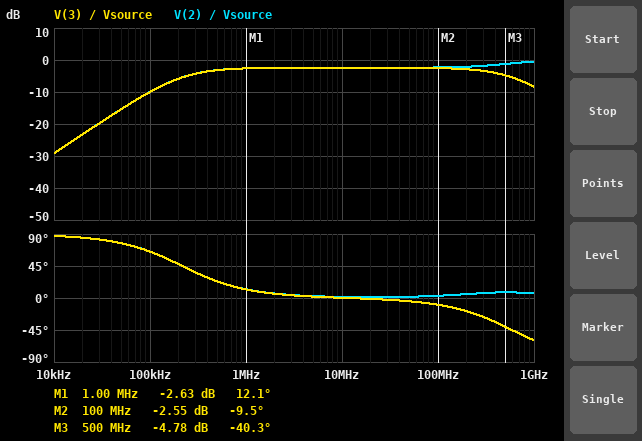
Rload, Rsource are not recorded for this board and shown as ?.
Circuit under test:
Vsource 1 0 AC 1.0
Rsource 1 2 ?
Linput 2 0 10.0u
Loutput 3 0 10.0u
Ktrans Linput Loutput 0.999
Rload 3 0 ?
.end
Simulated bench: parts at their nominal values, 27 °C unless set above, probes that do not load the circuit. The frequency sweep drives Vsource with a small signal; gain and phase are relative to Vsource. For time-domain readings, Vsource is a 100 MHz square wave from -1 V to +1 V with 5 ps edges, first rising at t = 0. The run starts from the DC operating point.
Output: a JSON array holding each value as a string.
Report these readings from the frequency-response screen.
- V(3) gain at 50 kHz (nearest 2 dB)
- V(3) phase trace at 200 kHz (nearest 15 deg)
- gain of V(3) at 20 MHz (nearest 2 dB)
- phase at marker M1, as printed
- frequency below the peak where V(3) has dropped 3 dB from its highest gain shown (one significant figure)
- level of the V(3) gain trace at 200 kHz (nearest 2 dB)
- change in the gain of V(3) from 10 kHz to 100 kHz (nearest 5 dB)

["-16 dB", "45 deg", "-2 dB", "12.1 deg", "200 kHz", "-6 dB", "20 dB"]
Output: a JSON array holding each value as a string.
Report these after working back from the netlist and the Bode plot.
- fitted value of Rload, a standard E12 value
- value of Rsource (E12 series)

["56 Ω", "18 Ω"]
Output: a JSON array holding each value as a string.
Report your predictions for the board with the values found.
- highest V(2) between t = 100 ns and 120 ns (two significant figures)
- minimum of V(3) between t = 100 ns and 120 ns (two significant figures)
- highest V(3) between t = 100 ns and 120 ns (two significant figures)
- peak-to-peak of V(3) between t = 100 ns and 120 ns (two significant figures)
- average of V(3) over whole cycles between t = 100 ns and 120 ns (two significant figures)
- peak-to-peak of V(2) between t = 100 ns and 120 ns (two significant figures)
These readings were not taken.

["1.9 V", "-110 mV", "1.4 V", "1.5 V", "650 mV", "2.5 V"]
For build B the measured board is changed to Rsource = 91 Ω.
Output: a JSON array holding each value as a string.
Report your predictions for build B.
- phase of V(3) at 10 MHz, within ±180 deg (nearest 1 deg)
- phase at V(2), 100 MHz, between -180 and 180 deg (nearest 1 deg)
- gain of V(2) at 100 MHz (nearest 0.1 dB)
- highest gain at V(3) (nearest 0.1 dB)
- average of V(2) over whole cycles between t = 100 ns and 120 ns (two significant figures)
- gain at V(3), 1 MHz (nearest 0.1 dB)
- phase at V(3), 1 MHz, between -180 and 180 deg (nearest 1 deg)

["3 deg", "8 deg", "-8.2 dB", "-8.4 dB", "260 mV", "-9.5 dB", "29 deg"]
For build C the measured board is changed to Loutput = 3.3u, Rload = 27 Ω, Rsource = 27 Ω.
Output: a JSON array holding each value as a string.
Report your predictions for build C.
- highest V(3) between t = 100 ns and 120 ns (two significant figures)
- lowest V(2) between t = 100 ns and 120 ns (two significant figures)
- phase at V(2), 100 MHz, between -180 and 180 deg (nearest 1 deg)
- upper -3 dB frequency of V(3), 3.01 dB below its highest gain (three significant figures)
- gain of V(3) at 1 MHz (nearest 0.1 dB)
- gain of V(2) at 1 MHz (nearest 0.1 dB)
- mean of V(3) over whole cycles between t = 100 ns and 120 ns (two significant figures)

["780 mV", "-650 mV", "2 deg", "867 MHz", "-7.7 dB", "-2.9 dB", "350 mV"]
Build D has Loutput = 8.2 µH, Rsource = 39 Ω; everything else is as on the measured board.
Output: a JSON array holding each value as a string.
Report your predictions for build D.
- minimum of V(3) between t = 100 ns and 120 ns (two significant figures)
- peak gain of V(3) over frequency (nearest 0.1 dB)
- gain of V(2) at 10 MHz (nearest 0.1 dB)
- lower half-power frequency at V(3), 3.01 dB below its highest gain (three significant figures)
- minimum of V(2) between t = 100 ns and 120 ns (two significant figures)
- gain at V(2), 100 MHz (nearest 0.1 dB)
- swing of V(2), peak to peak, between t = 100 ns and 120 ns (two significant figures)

["-150 mV", "-4.8 dB", "-3.9 dB", "395 kHz", "-880 mV", "-3.8 dB", "2.7 V"]
